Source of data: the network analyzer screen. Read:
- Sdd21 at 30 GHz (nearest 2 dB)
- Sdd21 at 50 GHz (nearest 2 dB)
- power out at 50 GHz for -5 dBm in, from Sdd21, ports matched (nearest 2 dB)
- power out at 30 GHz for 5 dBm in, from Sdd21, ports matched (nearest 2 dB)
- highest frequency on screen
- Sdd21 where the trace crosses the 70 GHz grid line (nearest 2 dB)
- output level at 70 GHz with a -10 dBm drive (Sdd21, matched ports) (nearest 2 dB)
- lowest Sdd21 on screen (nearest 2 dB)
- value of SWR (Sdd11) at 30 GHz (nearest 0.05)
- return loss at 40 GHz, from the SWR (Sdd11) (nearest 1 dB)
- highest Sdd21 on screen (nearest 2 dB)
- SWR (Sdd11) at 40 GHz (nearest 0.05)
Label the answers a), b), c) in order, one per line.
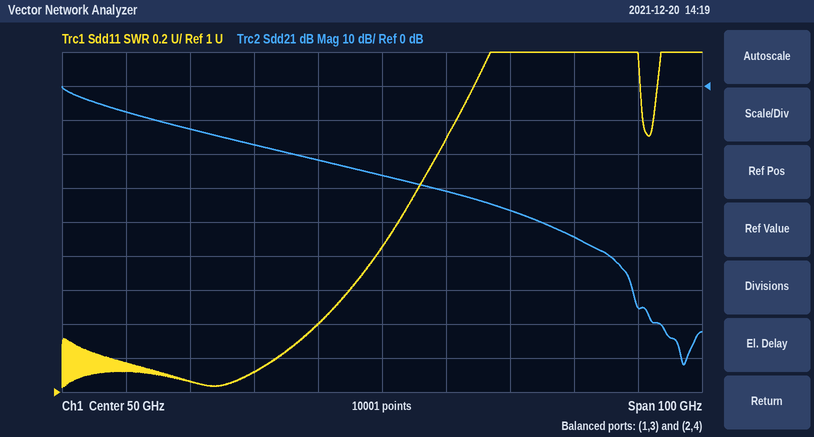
a) -18 dB
b) -26 dB
c) -32 dBm
d) -12 dBm
e) 100 GHz
f) -36 dB
g) -46 dBm
h) -82 dB
i) 1.10
j) 16 dB
k) 0 dB
l) 1.40
